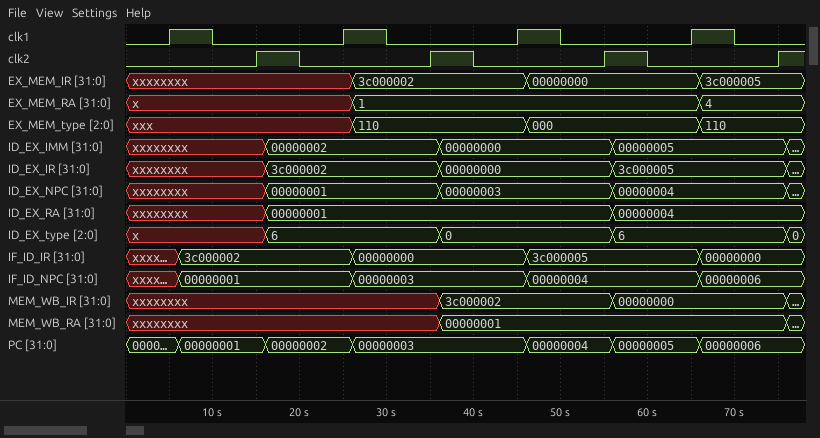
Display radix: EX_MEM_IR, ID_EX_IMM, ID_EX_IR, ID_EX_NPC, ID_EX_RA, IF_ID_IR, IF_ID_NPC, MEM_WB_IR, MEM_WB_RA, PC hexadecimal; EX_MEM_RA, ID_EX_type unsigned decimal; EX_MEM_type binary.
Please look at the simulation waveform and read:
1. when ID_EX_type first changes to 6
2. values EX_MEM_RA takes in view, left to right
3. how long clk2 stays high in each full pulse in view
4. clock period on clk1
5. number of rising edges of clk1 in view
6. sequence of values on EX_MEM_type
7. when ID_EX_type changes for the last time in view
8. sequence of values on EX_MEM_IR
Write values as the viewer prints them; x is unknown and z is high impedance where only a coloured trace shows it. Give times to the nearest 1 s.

16 s
x, 1, 4
5 s, 5 s, 5 s
20 s
4
xxx, 110, 000, 110
76 s
xxxxxxxx, 3c000002, 00000000, 3c000005
